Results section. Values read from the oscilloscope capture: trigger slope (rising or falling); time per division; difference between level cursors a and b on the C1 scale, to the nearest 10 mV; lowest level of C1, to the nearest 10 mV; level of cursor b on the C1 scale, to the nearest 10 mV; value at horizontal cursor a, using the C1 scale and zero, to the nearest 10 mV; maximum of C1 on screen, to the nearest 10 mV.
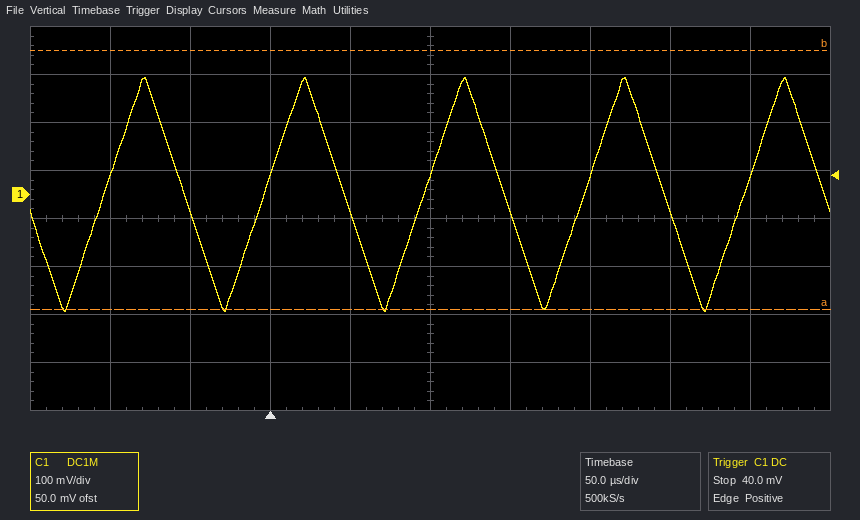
rising
50 µs
540 mV
-240 mV
300 mV
-240 mV
240 mV
